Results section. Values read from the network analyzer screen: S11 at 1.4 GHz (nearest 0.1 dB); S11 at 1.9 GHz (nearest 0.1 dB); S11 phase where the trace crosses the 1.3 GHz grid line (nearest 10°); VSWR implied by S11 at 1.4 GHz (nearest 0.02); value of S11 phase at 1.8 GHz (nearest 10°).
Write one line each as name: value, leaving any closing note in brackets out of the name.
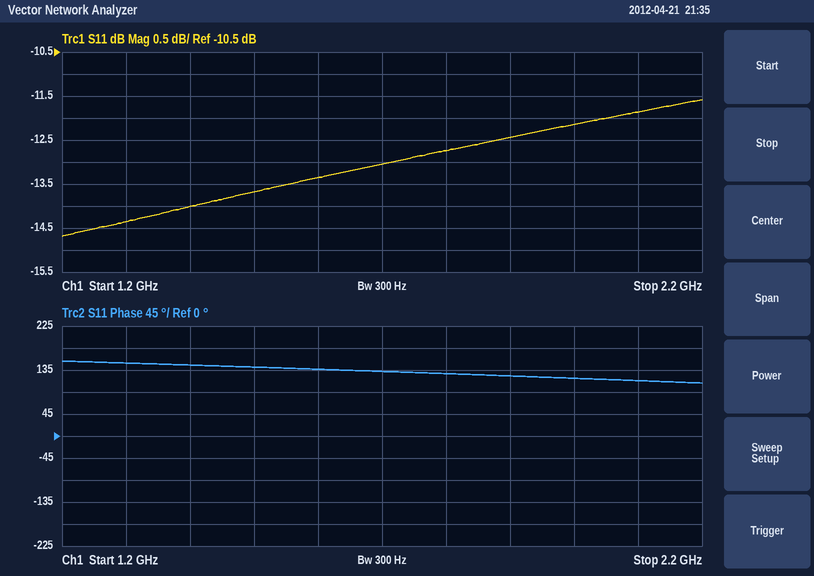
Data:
S11 at 1.4 GHz: -14.0 dB
S11 at 1.9 GHz: -12.4 dB
S11 phase where the trace crosses the 1.3 GHz grid line: 150°
VSWR implied by S11 at 1.4 GHz: 1.50
value of S11 phase at 1.8 GHz: 130°
